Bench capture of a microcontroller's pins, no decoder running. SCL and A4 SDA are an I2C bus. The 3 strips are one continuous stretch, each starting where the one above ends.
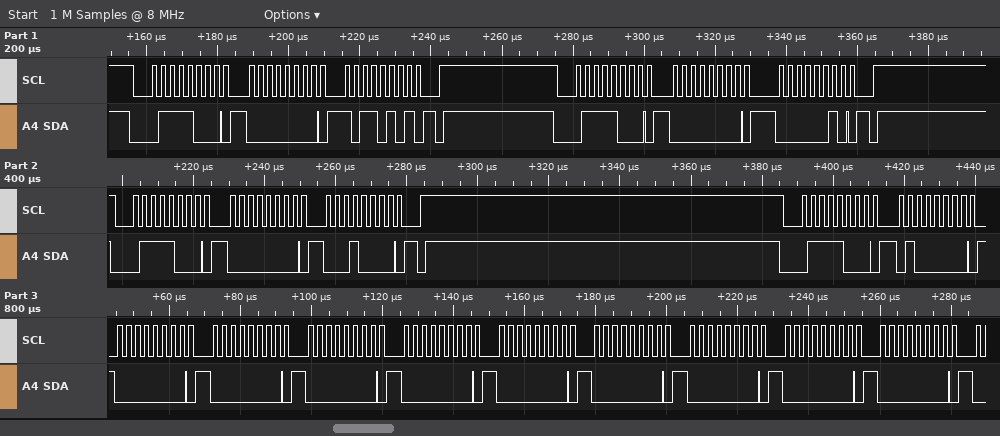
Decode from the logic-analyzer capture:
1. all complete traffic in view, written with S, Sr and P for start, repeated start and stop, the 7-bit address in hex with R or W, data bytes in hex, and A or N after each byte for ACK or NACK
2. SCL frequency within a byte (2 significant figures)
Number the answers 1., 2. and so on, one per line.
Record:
1. S 3CW A 00 A B5 A P S 3CW A 00 A 02 A P S 3CW A 00 A 10 A P S 3CW A 40 A 00 A 00 A 00 A 00 A 00 A 00 A 00 A 00 A 00 A
2. 400 kHz
